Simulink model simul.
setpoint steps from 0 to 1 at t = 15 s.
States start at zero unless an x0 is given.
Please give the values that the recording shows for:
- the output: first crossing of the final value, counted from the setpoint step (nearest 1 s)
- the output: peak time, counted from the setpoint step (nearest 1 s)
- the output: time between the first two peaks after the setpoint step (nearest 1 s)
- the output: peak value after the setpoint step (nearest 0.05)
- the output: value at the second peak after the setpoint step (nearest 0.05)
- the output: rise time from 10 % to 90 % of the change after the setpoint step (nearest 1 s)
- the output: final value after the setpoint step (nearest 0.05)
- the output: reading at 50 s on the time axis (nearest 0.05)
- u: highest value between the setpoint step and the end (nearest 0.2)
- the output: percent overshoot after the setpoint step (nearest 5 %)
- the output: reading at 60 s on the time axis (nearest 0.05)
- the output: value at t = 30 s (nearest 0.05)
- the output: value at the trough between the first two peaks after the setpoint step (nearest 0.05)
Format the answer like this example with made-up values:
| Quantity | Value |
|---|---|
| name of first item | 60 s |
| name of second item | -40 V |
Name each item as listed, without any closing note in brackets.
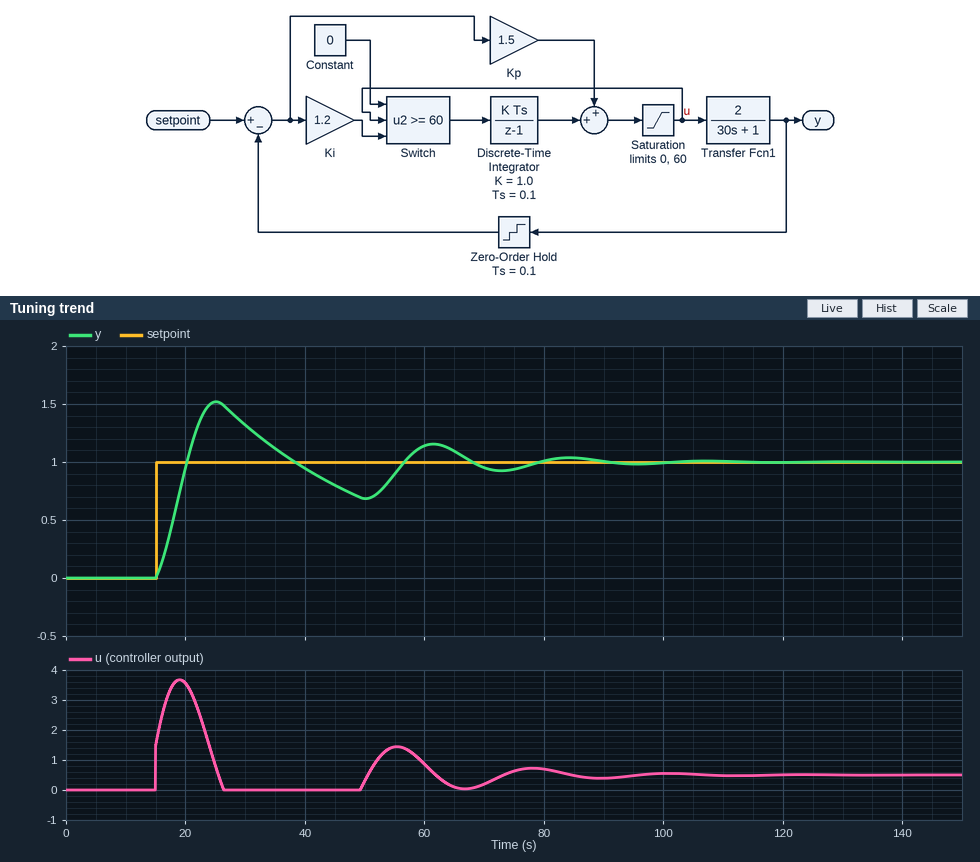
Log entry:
| Quantity | Value |
|---|---|
| the output: first crossing of the final value, counted from the setpoint step | 5 s |
| the output: peak time, counted from the setpoint step | 10 s |
| the output: time between the first two peaks after the setpoint step | 36 s |
| the output: peak value after the setpoint step | 1.50 |
| the output: value at the second peak after the setpoint step | 1.15 |
| the output: rise time from 10 % to 90 % of the change after the setpoint step | 4 s |
| the output: final value after the setpoint step | 1.00 |
| the output: reading at 50 s on the time axis | 0.70 |
| u: highest value between the setpoint step and the end | 3.6 |
| the output: percent overshoot after the setpoint step | 50 % |
| the output: reading at 60 s on the time axis | 1.15 |
| the output: value at t = 30 s | 1.30 |
| the output: value at the trough between the first two peaks after the setpoint step | 0.70 |
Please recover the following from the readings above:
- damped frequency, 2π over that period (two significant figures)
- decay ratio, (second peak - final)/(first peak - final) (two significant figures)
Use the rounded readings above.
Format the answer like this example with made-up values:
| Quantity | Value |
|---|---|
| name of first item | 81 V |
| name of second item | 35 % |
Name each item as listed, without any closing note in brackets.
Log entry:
| Quantity | Value |
|---|---|
| damped frequency, 2π over that period | 0.17 rad/s |
| decay ratio, (second peak - final)/(first peak - final) | 0.30 |
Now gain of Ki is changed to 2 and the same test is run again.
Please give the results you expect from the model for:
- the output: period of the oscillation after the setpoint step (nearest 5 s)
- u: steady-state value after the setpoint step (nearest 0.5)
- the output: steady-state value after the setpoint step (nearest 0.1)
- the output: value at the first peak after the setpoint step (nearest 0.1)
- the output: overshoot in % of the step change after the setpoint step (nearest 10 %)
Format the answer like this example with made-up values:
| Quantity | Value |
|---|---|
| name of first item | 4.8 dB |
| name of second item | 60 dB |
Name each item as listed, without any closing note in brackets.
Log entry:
| Quantity | Value |
|---|---|
| the output: period of the oscillation after the setpoint step | 40 s |
| u: steady-state value after the setpoint step | 0.5 |
| the output: steady-state value after the setpoint step | 1.0 |
| the output: value at the first peak after the setpoint step | 1.6 |
| the output: overshoot in % of the step change after the setpoint step | 60 % |
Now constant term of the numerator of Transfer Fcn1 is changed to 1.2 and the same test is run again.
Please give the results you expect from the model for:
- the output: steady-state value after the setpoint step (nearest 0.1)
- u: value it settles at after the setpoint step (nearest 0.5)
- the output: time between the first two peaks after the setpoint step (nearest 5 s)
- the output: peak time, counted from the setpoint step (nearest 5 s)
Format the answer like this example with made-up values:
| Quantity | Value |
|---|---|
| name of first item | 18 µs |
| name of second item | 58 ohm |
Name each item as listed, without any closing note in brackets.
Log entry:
| Quantity | Value |
|---|---|
| the output: steady-state value after the setpoint step | 1.0 |
| u: value it settles at after the setpoint step | 1.0 |
| the output: time between the first two peaks after the setpoint step | 40 s |
| the output: peak time, counted from the setpoint step | 15 s |
